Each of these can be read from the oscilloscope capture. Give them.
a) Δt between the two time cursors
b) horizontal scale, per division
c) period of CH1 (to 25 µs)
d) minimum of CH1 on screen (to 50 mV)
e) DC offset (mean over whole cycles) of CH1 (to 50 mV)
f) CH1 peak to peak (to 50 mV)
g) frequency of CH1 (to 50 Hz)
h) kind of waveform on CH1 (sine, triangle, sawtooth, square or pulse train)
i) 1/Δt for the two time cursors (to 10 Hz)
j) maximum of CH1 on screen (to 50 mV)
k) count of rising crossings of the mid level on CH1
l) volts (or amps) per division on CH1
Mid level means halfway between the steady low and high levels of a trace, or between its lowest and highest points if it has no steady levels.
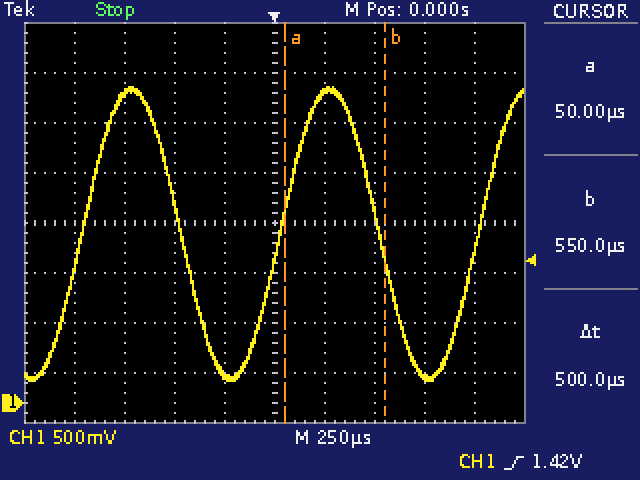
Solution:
500 µs
250 µs
1.000 ms
200 mV
1.70 V
2.95 V
1.00 kHz
sine
2.00 kHz
3.15 V
3
500 mV
